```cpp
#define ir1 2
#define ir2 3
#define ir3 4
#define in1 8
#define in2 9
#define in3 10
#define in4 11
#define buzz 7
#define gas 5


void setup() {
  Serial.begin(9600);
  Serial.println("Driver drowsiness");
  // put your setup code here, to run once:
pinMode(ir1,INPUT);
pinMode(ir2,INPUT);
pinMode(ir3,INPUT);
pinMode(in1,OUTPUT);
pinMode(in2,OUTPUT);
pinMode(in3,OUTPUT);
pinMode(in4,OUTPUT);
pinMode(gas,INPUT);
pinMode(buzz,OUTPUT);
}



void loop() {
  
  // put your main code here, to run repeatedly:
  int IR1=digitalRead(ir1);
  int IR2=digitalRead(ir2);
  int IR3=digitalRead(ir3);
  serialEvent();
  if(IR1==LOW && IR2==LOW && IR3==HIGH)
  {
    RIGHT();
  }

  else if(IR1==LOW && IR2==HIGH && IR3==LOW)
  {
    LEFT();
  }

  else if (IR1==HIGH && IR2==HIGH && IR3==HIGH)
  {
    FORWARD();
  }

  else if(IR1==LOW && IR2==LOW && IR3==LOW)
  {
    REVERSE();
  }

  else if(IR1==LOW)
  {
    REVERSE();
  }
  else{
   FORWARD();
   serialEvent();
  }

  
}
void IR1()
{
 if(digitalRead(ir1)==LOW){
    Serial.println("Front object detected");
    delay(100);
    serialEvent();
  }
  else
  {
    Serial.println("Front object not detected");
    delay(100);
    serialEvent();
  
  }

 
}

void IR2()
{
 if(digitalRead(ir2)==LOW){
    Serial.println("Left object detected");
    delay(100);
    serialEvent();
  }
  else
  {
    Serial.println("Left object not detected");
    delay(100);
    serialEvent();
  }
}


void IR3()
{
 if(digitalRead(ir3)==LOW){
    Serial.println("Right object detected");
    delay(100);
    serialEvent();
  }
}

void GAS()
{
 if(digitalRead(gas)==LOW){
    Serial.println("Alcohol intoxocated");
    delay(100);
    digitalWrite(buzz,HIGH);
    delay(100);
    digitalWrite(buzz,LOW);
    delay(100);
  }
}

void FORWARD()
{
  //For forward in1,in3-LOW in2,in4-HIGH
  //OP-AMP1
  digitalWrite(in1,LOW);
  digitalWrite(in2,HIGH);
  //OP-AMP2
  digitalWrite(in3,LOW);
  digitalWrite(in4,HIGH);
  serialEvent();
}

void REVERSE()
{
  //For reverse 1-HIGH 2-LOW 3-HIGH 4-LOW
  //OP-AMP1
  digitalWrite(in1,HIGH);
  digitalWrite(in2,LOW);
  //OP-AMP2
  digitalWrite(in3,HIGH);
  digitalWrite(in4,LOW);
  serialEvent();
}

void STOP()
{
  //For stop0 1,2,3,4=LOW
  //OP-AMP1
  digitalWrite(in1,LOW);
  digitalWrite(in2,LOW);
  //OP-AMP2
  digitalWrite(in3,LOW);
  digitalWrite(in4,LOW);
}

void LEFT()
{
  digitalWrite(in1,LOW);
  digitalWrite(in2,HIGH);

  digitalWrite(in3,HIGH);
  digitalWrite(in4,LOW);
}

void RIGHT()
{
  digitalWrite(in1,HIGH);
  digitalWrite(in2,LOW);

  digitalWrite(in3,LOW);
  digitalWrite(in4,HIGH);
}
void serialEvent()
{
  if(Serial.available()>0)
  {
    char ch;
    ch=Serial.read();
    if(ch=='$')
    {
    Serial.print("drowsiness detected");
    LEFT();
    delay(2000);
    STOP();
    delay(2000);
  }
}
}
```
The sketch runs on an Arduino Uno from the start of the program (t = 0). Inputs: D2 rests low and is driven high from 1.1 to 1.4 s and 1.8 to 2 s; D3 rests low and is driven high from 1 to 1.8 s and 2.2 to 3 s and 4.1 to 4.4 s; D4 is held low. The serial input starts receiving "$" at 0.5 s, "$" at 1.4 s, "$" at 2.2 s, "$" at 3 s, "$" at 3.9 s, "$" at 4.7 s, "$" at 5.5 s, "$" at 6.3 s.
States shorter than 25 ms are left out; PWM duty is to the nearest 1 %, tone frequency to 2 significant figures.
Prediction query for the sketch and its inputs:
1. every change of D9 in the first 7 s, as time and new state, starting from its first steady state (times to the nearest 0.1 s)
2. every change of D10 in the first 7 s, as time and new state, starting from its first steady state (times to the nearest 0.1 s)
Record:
0 s low; 0.5 s high; 2.5 s low; 4.5 s high; 6.5 s low
0 s high; 2.5 s low; 4.5 s high; 6.5 s low
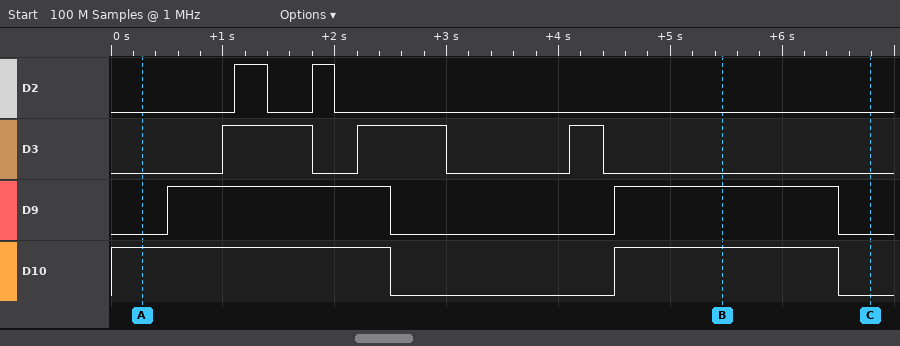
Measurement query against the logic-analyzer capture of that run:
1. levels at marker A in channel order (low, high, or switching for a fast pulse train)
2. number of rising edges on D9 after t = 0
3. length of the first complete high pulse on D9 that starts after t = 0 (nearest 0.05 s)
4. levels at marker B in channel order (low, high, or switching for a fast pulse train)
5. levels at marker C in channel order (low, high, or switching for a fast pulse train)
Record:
D2 low, D3 low, D9 low, D10 high
2
2.00 s
D2 low, D3 low, D9 high, D10 high
D2 low, D3 low, D9 low, D10 low
